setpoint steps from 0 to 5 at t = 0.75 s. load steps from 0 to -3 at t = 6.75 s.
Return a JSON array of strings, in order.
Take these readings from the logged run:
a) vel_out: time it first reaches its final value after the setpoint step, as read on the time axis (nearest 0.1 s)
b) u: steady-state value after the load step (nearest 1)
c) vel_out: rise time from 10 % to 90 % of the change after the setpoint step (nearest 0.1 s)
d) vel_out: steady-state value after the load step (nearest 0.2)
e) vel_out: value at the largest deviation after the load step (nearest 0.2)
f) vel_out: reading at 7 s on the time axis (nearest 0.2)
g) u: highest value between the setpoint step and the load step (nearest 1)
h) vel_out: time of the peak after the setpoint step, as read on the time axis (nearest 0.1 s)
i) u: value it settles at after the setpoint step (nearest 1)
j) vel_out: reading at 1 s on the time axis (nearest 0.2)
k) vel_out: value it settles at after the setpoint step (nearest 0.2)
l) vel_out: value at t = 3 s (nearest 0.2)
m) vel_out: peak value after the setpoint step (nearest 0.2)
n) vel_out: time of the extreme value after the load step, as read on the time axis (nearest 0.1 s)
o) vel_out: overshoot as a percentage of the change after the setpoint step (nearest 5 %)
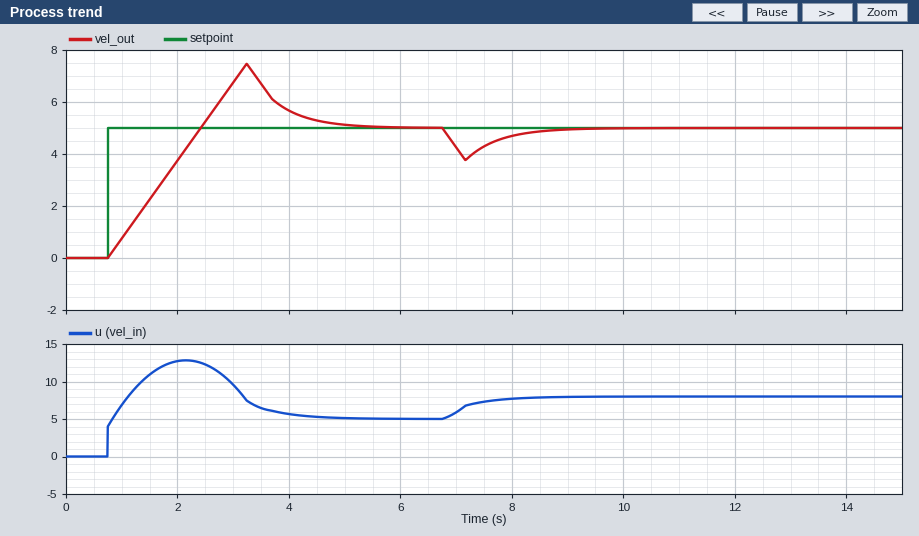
["2.4 s", "8", "1.3 s", "5.0", "3.8", "4.2", "13", "3.2 s", "5", "0.8", "5.0", "6.8", "7.4", "7.2 s", "50 %"]
